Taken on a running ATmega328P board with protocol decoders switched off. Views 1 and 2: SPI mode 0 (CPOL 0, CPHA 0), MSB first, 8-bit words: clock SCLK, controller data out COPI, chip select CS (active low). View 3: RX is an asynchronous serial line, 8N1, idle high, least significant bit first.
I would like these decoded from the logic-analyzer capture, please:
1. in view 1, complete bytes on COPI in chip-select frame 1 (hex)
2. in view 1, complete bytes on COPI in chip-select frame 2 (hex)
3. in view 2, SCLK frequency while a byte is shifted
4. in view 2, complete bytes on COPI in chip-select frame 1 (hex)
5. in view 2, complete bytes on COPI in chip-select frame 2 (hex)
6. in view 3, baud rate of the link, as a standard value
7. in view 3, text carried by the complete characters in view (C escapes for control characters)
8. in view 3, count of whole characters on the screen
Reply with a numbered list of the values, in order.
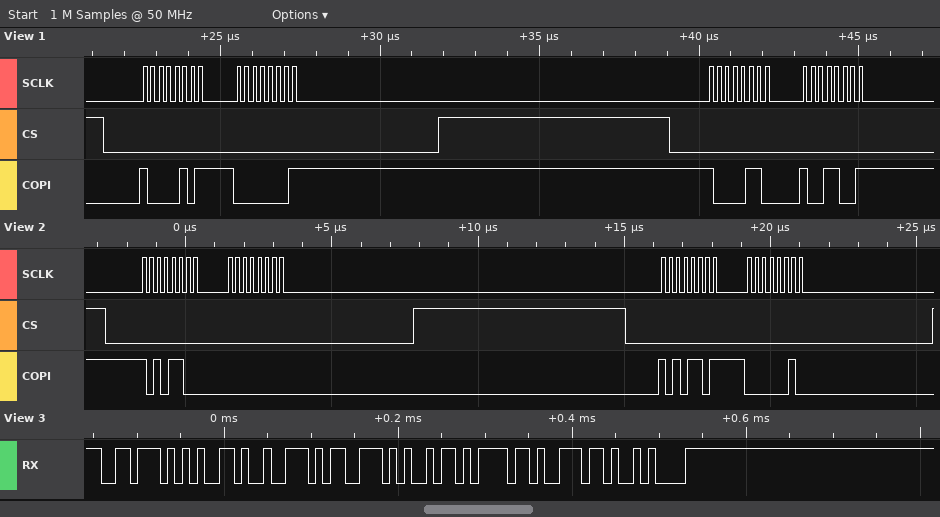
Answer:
1. 85 01
2. 86 99
3. 4 MHz
4. AC 00
5. AD 02
6. 115200 baud
7. "version\n"
8. 8
